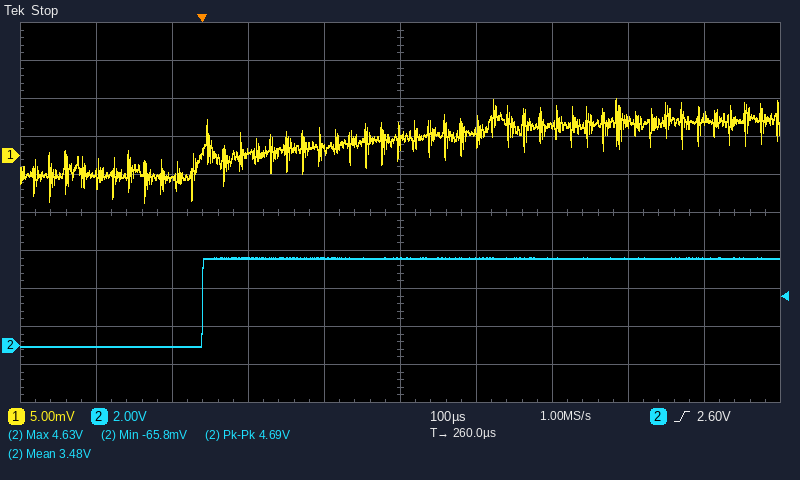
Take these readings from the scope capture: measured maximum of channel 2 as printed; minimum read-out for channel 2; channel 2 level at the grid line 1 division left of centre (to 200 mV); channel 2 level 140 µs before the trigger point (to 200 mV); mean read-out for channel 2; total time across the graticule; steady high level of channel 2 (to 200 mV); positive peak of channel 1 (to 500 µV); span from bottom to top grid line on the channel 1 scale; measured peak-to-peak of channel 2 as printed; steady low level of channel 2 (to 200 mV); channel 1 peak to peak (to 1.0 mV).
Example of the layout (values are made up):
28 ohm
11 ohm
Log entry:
4.63 V
-65.8 mV
4.6 V
0.0 V
3.48 V
1 ms
4.6 V
7.5 mV
50 mV
4.69 V
0.0 V
14.0 mV
